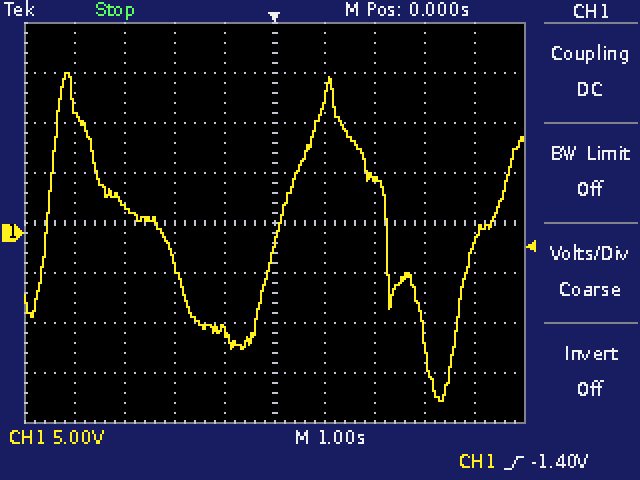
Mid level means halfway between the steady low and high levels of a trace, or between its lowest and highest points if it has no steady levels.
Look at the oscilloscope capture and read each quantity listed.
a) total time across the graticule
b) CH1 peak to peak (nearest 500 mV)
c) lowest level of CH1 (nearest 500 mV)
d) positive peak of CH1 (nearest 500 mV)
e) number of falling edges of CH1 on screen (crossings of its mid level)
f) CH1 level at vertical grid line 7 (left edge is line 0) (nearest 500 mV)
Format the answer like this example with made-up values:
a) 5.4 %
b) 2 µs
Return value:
a) 10 s
b) 33.0 V
c) -17.0 V
d) 16.0 V
e) 2
f) 5.5 V
